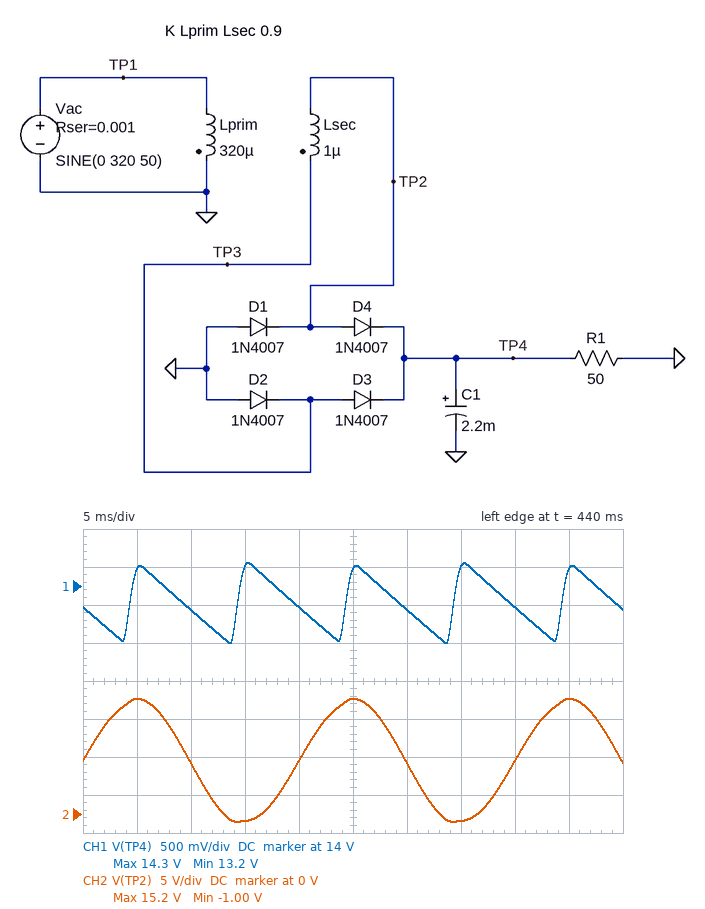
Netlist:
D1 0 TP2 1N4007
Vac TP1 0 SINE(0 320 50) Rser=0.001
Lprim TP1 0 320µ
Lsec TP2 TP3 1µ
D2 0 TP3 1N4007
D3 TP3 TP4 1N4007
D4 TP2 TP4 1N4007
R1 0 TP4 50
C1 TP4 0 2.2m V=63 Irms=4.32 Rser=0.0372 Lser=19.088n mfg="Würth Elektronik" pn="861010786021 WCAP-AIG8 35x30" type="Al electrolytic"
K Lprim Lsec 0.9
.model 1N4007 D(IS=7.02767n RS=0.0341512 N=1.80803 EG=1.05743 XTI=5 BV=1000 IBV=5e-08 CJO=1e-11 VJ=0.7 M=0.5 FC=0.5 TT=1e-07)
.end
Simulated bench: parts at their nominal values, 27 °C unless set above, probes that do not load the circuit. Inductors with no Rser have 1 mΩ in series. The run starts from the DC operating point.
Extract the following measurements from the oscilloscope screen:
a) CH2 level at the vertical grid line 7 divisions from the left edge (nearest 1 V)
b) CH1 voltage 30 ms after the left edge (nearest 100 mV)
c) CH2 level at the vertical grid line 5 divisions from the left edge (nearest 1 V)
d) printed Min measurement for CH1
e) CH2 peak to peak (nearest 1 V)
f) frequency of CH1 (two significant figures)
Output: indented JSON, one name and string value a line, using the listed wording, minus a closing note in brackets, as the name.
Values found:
{
  "CH2 level at the vertical grid line 7 divisions from the left edge": "-1 V",
  "CH1 voltage 30 ms after the left edge": "13.7 V",
  "CH2 level at the vertical grid line 5 divisions from the left edge": "15 V",
  "printed Min measurement for CH1": "13.2 V",
  "CH2 peak to peak": "16 V",
  "frequency of CH1": "100 Hz"
}
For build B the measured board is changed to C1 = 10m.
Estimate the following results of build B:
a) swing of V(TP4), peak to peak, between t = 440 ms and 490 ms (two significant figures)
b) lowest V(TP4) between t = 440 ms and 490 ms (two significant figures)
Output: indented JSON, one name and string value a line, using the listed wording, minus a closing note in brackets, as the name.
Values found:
{
  "swing of V(TP4), peak to peak, between t = 440 ms and 490 ms": "280 mV",
  "lowest V(TP4) between t = 440 ms and 490 ms": "14 V"
}
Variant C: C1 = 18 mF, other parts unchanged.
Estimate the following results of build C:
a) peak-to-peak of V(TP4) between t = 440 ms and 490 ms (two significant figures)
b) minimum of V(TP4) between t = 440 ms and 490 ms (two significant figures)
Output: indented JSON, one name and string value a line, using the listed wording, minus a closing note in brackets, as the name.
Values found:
{
  "peak-to-peak of V(TP4) between t = 440 ms and 490 ms": "190 mV",
  "minimum of V(TP4) between t = 440 ms and 490 ms": "14 V"
}
